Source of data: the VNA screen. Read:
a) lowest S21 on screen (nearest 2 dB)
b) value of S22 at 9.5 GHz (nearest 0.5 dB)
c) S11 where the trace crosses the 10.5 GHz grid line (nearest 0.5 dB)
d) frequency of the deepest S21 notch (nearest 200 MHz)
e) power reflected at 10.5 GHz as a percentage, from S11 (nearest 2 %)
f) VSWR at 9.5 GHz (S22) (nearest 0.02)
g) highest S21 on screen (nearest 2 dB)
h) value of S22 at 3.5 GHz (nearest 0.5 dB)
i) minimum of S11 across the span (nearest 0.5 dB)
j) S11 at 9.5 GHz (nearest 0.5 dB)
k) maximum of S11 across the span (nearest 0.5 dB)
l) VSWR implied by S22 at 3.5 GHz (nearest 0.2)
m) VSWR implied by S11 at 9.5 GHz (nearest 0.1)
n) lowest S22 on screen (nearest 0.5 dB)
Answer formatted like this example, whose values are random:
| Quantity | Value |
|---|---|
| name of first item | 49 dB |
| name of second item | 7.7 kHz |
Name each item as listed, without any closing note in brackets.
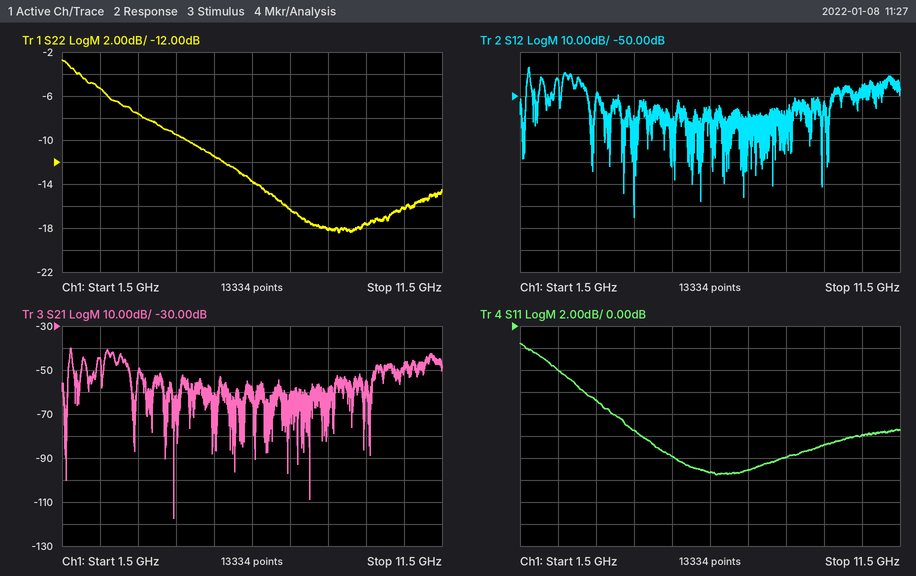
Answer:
| Quantity | Value |
|---|---|
| lowest S21 on screen | -118 dB |
| value of S22 at 9.5 GHz | -17.5 dB |
| S11 where the trace crosses the 10.5 GHz grid line | -10.0 dB |
| frequency of the deepest S21 notch | 4.4 GHz |
| power reflected at 10.5 GHz as a percentage, from S11 | 10 % |
| VSWR at 9.5 GHz (S22) | 1.30 |
| highest S21 on screen | -40 dB |
| value of S22 at 3.5 GHz | -7.5 dB |
| minimum of S11 across the span | -13.5 dB |
| S11 at 9.5 GHz | -11.0 dB |
| maximum of S11 across the span | -1.5 dB |
| VSWR implied by S22 at 3.5 GHz | 2.4 |
| VSWR implied by S11 at 9.5 GHz | 1.8 |
| lowest S22 on screen | -18.5 dB |
